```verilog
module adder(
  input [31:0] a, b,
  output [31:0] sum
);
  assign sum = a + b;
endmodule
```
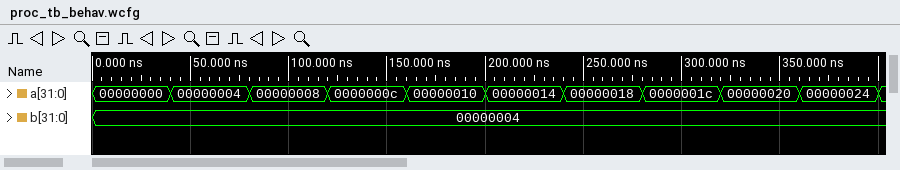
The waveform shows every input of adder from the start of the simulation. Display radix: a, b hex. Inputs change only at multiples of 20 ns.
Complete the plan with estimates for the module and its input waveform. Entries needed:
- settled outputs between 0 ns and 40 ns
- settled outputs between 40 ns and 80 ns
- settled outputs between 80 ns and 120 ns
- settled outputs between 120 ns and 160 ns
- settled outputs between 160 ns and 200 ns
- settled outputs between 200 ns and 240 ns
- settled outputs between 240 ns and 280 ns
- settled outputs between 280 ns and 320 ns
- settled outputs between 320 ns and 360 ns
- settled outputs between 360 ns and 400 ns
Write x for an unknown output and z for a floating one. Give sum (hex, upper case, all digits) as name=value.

sum=00000004
sum=00000008
sum=0000000C
sum=00000010
sum=00000014
sum=00000018
sum=0000001C
sum=00000020
sum=00000024
sum=00000028
